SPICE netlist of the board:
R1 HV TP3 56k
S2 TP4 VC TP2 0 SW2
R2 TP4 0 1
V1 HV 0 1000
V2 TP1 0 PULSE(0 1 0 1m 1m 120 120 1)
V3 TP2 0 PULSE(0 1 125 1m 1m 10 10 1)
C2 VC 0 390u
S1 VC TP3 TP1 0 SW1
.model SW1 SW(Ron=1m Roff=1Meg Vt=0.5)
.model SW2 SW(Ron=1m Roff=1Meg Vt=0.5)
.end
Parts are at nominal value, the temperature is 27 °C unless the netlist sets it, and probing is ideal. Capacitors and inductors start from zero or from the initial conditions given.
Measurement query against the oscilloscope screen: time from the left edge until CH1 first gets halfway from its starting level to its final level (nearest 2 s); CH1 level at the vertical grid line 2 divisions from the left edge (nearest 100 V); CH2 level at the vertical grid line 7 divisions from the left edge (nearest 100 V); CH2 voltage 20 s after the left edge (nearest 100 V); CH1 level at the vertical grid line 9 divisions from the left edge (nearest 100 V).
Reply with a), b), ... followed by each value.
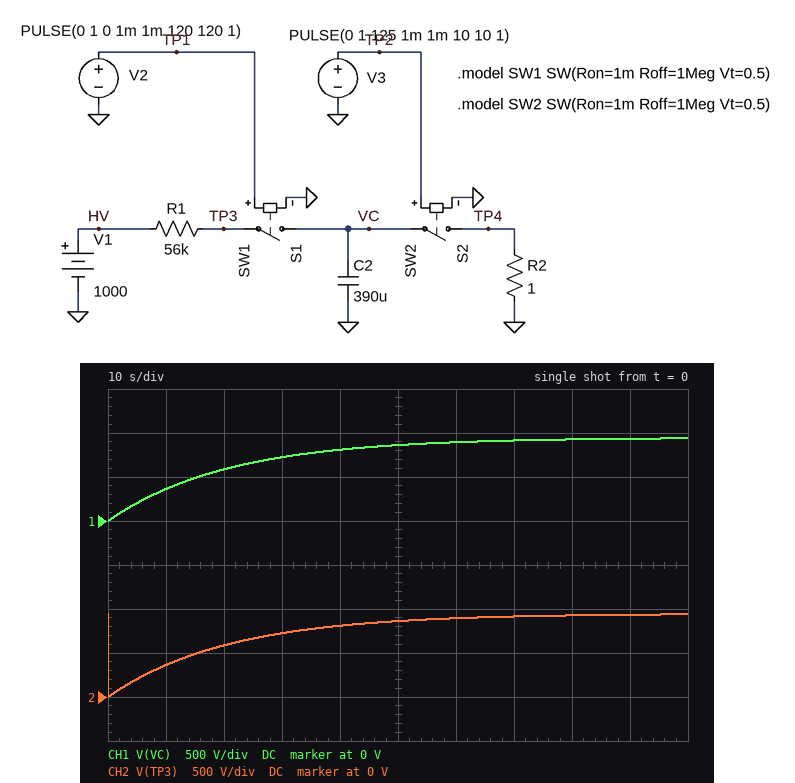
a) 14 s
b) 600 V
c) 900 V
d) 600 V
e) 900 V
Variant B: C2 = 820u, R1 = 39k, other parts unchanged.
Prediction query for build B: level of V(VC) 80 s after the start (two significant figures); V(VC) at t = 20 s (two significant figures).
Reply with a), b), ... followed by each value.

a) 890 V
b) 460 V
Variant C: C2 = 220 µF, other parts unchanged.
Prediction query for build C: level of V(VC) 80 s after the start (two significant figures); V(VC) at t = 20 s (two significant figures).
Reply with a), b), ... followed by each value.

a) 950 V
b) 780 V
